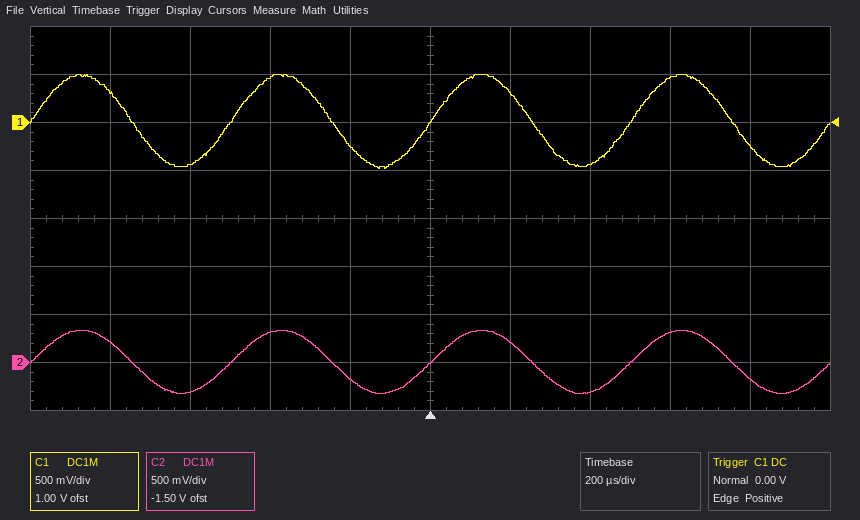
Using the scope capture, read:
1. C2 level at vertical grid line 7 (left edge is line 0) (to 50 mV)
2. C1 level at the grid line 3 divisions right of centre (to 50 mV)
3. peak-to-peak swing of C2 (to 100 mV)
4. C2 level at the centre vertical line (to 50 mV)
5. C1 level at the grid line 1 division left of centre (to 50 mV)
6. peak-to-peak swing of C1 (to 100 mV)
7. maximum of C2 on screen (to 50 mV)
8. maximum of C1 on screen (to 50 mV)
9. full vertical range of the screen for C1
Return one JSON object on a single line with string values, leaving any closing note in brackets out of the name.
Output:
{"C2 level at vertical grid line 7 (left edge is line 0)": "-300 mV", "C1 level at the grid line 3 divisions right of centre": "450 mV", "peak-to-peak swing of C2": "700 mV", "C2 level at the centre vertical line": "0 mV", "C1 level at the grid line 1 division left of centre": "-250 mV", "peak-to-peak swing of C1": "1.00 V", "maximum of C2 on screen": "350 mV", "maximum of C1 on screen": "500 mV", "full vertical range of the screen for C1": "4 V"}
